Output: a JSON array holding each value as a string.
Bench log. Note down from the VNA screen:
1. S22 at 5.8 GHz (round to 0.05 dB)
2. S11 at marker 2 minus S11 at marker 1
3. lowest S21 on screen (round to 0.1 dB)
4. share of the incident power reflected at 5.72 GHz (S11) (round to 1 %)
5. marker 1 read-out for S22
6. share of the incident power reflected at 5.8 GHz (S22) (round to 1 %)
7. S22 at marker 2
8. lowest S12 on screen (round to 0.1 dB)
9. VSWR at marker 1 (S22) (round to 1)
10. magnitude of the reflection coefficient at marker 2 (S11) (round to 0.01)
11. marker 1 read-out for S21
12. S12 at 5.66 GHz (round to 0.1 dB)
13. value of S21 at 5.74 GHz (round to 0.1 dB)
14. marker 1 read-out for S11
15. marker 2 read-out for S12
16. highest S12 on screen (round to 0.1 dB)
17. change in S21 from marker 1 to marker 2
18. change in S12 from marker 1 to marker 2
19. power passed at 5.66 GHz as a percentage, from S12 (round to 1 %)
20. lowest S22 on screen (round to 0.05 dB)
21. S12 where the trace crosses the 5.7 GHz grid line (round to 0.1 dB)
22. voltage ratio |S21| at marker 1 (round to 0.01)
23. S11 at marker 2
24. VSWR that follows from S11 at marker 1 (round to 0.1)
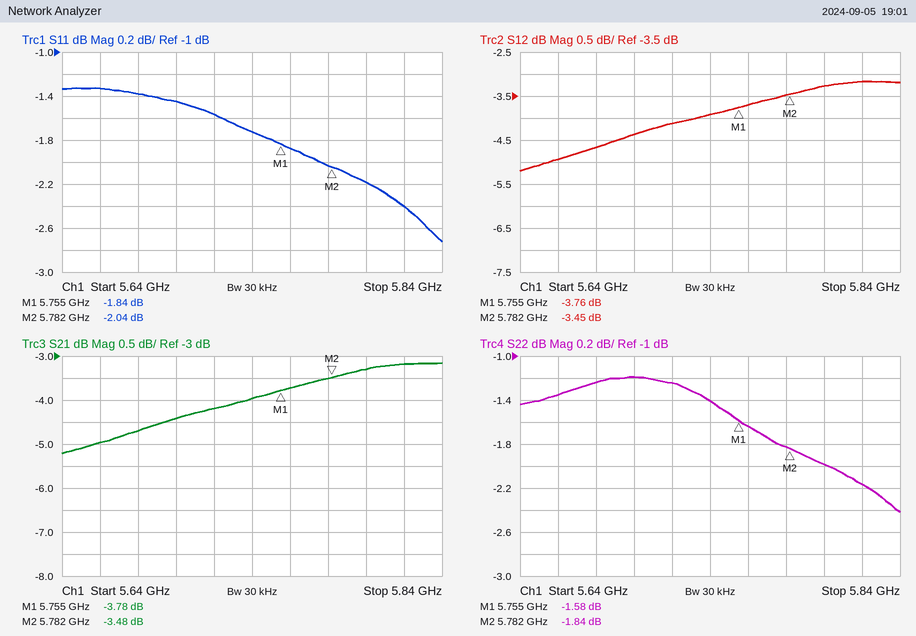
["-2.00 dB", "-0.20 dB", "-5.2 dB", "70 %", "-1.58 dB", "63 %", "-1.84 dB", "-5.2 dB", "11", "0.79", "-3.78 dB", "-4.9 dB", "-4.0 dB", "-1.84 dB", "-3.45 dB", "-3.2 dB", "0.30 dB", "0.31 dB", "32 %", "-2.40 dB", "-4.4 dB", "0.65", "-2.04 dB", "9.5"]
